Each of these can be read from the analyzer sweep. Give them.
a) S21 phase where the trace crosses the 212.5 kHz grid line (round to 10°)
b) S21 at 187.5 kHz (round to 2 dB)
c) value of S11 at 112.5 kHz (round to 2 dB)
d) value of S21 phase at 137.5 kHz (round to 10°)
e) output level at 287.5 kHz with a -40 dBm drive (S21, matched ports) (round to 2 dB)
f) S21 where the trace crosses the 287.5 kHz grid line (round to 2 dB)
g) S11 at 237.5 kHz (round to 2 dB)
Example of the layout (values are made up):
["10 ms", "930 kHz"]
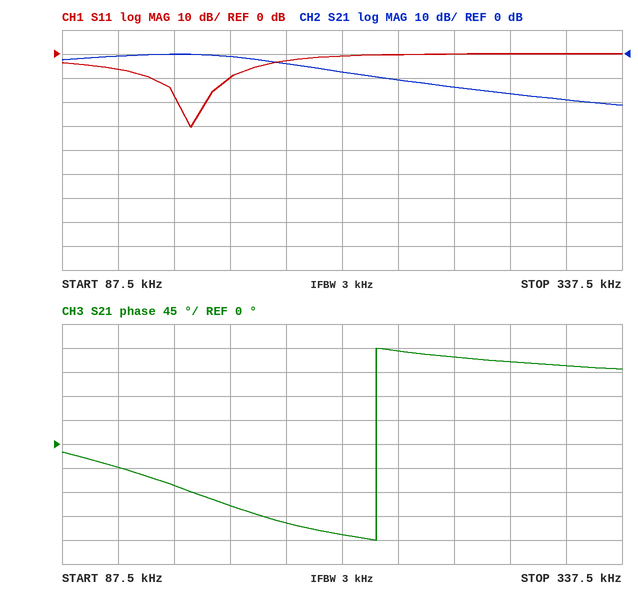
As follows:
["-170°", "-4 dB", "-6 dB", "-80°", "-56 dBm", "-16 dB", "0 dB"]
